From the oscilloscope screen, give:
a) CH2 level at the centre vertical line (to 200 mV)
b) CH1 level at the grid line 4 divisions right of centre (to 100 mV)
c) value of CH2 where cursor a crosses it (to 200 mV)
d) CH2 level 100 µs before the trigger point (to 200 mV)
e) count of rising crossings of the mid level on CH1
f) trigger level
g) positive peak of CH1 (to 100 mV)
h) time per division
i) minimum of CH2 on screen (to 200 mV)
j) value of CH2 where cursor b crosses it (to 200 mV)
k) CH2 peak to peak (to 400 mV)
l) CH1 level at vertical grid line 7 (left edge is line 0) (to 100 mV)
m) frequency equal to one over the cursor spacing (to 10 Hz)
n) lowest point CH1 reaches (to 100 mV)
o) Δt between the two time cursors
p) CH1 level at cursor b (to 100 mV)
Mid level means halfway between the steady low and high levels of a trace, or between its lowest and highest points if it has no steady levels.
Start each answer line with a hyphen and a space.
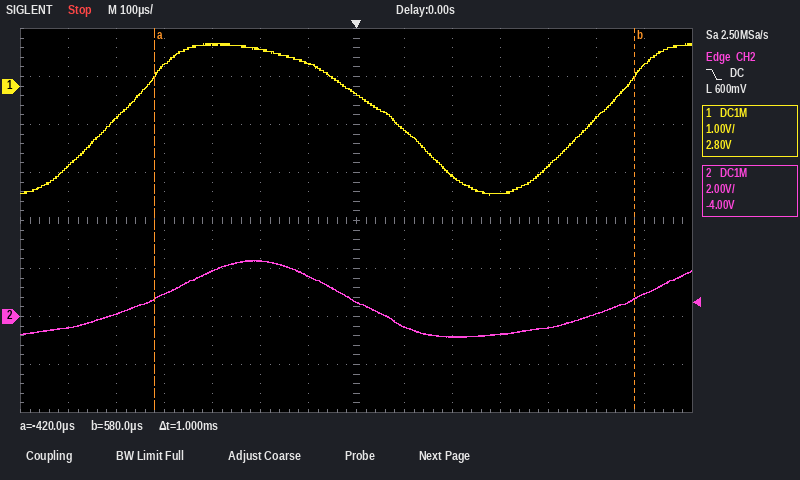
- 600 mV
- -1.7 V
- 800 mV
- 1.6 V
- 2
- 600 mV
- 900 mV
- 100 µs
- -800 mV
- 800 mV
- 3.2 V
- -200 mV
- 1.00 kHz
- -2.3 V
- 1 ms
- 200 mV
